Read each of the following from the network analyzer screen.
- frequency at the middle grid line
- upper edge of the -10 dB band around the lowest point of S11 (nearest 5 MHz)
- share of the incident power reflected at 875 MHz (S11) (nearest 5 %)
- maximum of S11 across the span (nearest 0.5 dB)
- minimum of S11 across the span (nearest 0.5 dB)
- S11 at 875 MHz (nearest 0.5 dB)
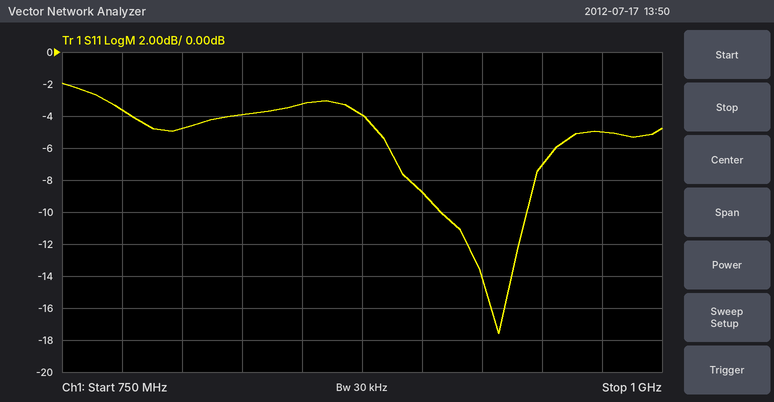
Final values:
875 MHz
945 MHz
40 %
-2.0 dB
-17.5 dB
-4.0 dB
